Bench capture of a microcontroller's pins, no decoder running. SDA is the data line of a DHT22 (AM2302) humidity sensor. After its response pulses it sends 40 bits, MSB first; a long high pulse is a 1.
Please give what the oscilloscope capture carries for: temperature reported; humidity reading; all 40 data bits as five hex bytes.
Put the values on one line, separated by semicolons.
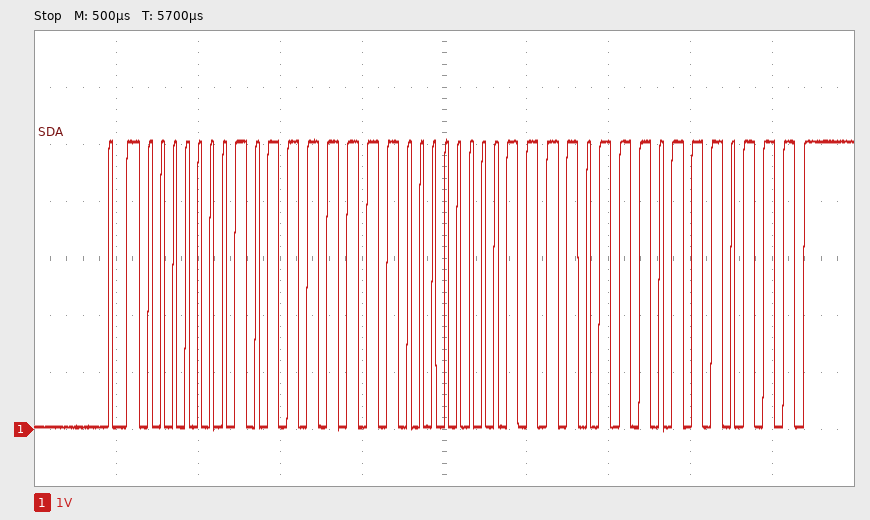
24.7 °C; 38.3 %; 01 7F 00 F7 77
